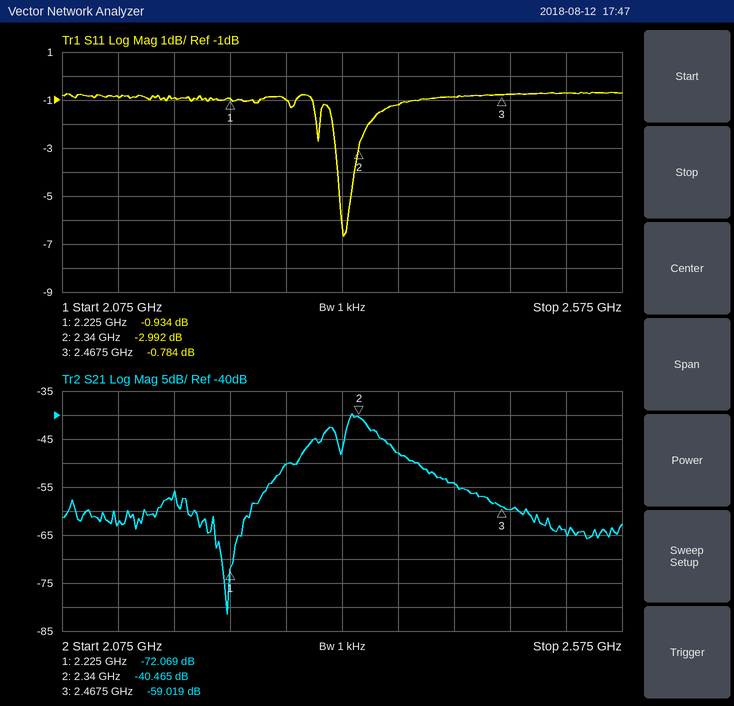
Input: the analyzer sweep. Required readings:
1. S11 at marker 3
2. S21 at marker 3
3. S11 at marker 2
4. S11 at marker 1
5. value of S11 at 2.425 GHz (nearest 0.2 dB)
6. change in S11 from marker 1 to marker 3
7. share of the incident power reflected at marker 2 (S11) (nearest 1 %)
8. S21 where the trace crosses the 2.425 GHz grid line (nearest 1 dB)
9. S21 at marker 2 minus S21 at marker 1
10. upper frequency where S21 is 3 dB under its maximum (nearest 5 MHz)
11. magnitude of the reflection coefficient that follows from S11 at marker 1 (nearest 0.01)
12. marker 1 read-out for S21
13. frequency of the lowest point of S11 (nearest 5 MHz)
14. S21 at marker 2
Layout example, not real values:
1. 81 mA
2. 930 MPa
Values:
1. -0.784 dB
2. -59.019 dB
3. -2.992 dB
4. -0.934 dB
5. -0.8 dB
6. 0.150 dB
7. 50 %
8. -54 dB
9. 31.604 dB
10. 2.350 GHz
11. 0.90
12. -72.069 dB
13. 2.325 GHz
14. -40.465 dB
